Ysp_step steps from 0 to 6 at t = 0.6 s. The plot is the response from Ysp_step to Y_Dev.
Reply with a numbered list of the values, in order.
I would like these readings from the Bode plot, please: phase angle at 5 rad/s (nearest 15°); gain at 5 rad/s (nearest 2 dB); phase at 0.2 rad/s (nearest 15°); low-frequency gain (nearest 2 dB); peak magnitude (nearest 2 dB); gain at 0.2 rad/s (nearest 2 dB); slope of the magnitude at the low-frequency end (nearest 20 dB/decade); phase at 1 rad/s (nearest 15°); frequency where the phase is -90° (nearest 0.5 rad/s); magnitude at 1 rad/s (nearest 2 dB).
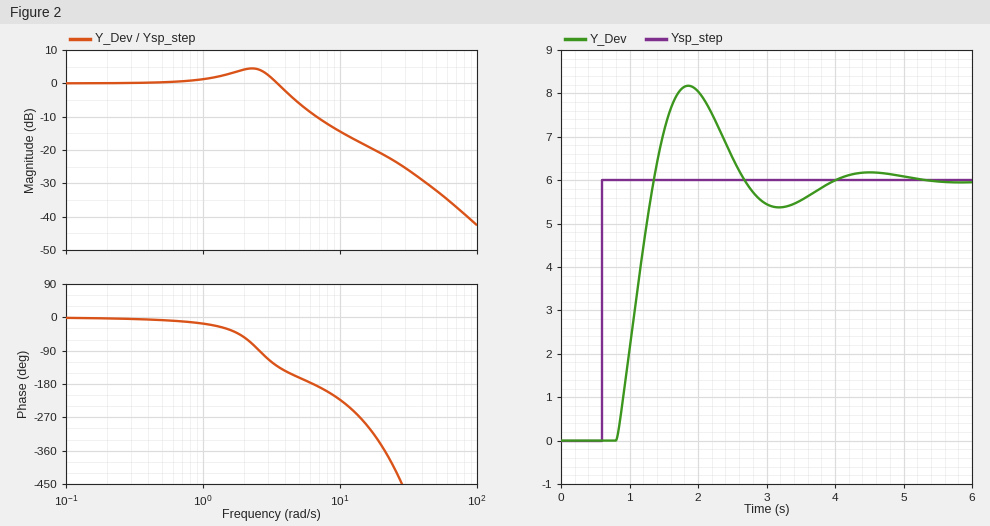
1. -165°
2. -6 dB
3. 0°
4. 0 dB
5. 4 dB
6. 0 dB
7. 0 dB/decade
8. -15°
9. 2.5 rad/s
10. 2 dB
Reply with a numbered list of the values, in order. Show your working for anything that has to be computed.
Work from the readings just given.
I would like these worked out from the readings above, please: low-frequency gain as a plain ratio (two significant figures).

1. 10^(0 / 20) = 1.0
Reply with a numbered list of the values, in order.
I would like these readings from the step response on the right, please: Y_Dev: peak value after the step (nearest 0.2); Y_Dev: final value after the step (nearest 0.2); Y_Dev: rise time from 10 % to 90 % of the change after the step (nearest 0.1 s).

1. 8.2
2. 6.0
3. 0.4 s
